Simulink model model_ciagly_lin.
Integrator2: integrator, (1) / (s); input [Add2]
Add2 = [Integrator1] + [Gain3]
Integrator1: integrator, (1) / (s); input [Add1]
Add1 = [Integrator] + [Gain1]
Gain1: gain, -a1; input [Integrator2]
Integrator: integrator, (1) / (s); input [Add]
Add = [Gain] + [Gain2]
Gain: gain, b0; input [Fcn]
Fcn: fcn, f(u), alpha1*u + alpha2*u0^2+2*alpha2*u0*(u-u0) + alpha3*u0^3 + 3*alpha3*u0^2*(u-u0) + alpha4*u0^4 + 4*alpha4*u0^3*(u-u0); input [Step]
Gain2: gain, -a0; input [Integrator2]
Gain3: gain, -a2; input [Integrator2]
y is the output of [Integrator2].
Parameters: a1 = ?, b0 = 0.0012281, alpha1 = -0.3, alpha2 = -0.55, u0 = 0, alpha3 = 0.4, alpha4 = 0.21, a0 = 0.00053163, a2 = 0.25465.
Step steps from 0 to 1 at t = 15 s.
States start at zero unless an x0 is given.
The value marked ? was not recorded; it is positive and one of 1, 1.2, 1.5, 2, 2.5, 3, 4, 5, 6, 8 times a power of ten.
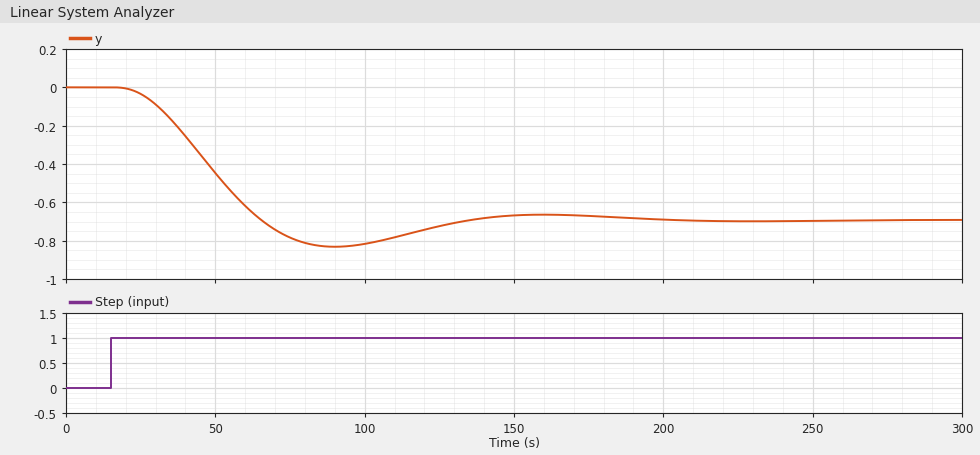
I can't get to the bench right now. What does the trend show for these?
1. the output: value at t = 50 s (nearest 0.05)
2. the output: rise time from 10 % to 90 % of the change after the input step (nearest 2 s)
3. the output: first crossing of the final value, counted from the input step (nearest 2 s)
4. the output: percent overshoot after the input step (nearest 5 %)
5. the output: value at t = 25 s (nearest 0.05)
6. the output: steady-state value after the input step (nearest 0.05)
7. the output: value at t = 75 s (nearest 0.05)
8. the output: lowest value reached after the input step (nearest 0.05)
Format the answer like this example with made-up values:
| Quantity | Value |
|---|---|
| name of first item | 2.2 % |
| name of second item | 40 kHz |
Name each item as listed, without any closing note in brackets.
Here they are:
| Quantity | Value |
|---|---|
| the output: value at t = 50 s | -0.45 |
| the output: rise time from 10 % to 90 % of the change after the input step | 32 s |
| the output: first crossing of the final value, counted from the input step | 50 s |
| the output: percent overshoot after the input step | 20 % |
| the output: value at t = 25 s | -0.05 |
| the output: steady-state value after the input step | -0.70 |
| the output: value at t = 75 s | -0.80 |
| the output: lowest value reached after the input step | -0.85 |
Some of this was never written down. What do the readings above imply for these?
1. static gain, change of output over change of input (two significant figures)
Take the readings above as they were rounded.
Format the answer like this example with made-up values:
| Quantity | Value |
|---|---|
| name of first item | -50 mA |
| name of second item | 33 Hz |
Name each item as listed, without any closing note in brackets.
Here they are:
| Quantity | Value |
|---|---|
| static gain, change of output over change of input | -0.70 |
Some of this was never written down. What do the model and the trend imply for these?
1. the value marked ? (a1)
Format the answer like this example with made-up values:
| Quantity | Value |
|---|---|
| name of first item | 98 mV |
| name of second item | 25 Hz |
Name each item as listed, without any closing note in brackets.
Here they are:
| Quantity | Value |
|---|---|
| the value marked ? | 0.012 |
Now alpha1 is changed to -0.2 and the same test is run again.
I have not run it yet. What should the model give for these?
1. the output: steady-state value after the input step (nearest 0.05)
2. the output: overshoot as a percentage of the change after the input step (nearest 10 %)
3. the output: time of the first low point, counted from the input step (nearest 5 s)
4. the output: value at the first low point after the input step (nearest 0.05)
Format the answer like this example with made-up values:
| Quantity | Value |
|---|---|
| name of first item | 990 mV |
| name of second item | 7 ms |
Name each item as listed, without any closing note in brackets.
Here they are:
| Quantity | Value |
|---|---|
| the output: steady-state value after the input step | -0.45 |
| the output: overshoot as a percentage of the change after the input step | 20 % |
| the output: time of the first low point, counted from the input step | 75 s |
| the output: value at the first low point after the input step | -0.55 |
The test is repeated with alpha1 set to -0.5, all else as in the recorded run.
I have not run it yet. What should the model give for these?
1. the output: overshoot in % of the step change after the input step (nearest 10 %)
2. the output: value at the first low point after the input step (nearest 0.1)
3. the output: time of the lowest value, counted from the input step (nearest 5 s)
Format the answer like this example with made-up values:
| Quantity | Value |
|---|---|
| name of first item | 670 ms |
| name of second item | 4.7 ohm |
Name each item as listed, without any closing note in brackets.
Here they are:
| Quantity | Value |
|---|---|
| the output: overshoot in % of the step change after the input step | 20 % |
| the output: value at the first low point after the input step | -1.4 |
| the output: time of the lowest value, counted from the input step | 75 s |
